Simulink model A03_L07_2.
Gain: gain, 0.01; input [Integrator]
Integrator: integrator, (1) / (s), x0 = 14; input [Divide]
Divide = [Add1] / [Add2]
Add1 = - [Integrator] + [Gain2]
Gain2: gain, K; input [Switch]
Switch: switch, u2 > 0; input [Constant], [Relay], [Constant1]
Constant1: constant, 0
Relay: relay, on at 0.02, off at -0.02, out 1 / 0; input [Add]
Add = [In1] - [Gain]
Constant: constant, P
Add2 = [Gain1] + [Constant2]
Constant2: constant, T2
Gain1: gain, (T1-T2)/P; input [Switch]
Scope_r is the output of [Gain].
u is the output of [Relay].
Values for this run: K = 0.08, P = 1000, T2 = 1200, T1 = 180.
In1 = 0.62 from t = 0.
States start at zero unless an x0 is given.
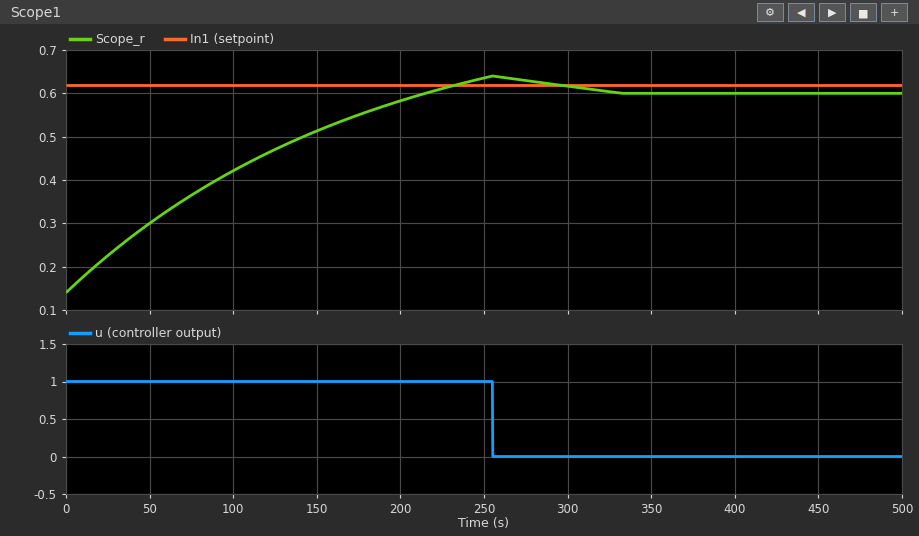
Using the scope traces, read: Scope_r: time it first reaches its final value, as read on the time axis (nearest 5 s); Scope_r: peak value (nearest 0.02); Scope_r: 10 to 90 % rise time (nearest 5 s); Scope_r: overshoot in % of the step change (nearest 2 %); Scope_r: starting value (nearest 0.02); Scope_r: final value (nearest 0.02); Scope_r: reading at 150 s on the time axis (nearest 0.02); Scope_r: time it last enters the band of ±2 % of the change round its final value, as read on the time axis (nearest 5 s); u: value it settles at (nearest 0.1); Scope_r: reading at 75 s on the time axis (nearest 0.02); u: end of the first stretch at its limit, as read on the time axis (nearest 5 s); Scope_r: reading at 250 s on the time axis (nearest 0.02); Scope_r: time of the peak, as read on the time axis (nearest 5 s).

215 s
0.64
165 s
8 %
0.14
0.60
0.52
315 s
0.0
0.36
255 s
0.64
255 s
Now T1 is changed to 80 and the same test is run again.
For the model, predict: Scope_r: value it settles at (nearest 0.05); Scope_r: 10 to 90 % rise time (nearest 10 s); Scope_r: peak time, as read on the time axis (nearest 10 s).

0.60
70 s
110 s
